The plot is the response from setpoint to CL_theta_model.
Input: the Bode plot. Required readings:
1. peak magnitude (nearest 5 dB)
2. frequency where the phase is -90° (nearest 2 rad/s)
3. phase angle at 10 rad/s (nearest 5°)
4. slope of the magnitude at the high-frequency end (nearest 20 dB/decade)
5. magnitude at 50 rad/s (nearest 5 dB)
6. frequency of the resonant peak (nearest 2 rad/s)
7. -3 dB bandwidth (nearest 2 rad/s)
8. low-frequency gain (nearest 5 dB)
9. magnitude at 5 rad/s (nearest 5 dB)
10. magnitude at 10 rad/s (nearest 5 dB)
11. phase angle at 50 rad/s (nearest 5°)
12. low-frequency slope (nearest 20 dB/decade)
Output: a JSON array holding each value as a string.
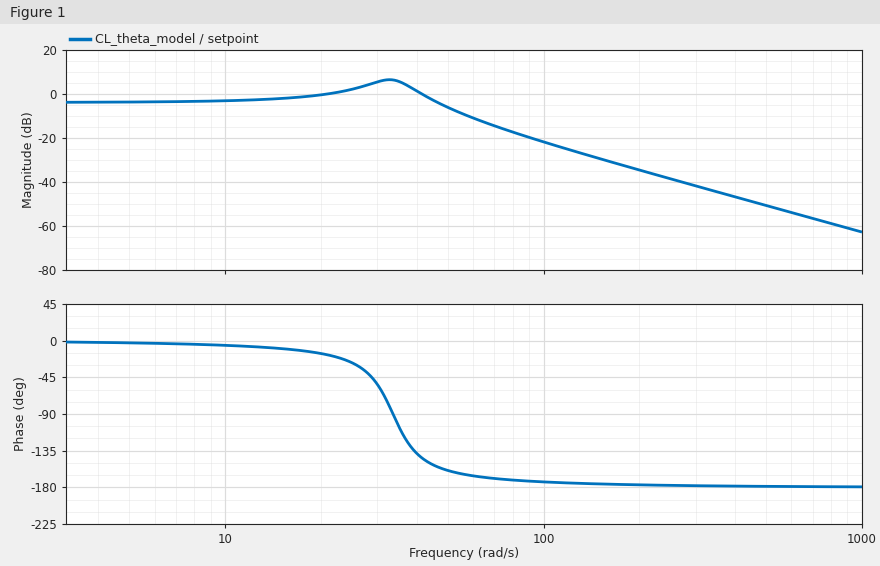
["5 dB", "34 rad/s", "-5°", "-40 dB/decade", "-5 dB", "32 rad/s", "52 rad/s", "-5 dB", "-5 dB", "-5 dB", "-160°", "0 dB/decade"]
